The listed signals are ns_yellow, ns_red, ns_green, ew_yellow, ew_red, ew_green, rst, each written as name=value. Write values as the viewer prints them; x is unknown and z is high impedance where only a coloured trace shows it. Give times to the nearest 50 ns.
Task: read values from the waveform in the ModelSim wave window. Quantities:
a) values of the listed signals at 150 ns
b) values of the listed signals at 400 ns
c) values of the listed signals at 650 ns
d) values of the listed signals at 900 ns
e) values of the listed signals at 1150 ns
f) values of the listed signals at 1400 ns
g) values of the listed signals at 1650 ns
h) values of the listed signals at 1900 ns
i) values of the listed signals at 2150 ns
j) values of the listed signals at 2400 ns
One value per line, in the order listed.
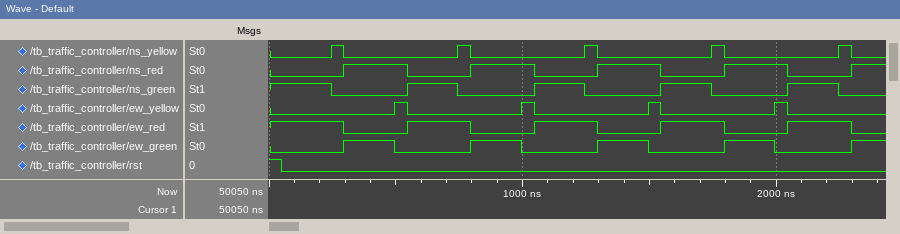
ns_yellow=0, ns_red=0, ns_green=1, ew_yellow=0, ew_red=1, ew_green=0, rst=0
ns_yellow=0, ns_red=1, ns_green=0, ew_yellow=0, ew_red=0, ew_green=1, rst=0
ns_yellow=0, ns_red=0, ns_green=1, ew_yellow=0, ew_red=1, ew_green=0, rst=0
ns_yellow=0, ns_red=1, ns_green=0, ew_yellow=0, ew_red=0, ew_green=1, rst=0
ns_yellow=0, ns_red=0, ns_green=1, ew_yellow=0, ew_red=1, ew_green=0, rst=0
ns_yellow=0, ns_red=1, ns_green=0, ew_yellow=0, ew_red=0, ew_green=1, rst=0
ns_yellow=0, ns_red=0, ns_green=1, ew_yellow=0, ew_red=1, ew_green=0, rst=0
ns_yellow=0, ns_red=1, ns_green=0, ew_yellow=0, ew_red=0, ew_green=1, rst=0
ns_yellow=0, ns_red=0, ns_green=1, ew_yellow=0, ew_red=1, ew_green=0, rst=0
ns_yellow=0, ns_red=1, ns_green=0, ew_yellow=0, ew_red=0, ew_green=1, rst=0
